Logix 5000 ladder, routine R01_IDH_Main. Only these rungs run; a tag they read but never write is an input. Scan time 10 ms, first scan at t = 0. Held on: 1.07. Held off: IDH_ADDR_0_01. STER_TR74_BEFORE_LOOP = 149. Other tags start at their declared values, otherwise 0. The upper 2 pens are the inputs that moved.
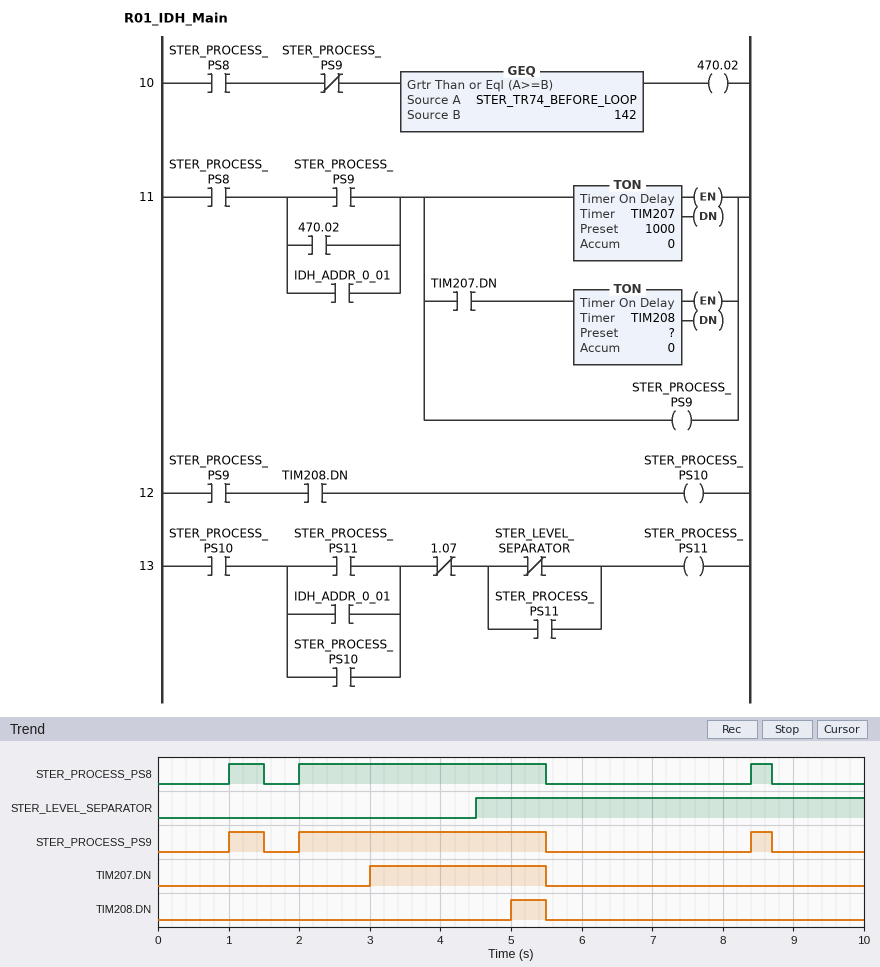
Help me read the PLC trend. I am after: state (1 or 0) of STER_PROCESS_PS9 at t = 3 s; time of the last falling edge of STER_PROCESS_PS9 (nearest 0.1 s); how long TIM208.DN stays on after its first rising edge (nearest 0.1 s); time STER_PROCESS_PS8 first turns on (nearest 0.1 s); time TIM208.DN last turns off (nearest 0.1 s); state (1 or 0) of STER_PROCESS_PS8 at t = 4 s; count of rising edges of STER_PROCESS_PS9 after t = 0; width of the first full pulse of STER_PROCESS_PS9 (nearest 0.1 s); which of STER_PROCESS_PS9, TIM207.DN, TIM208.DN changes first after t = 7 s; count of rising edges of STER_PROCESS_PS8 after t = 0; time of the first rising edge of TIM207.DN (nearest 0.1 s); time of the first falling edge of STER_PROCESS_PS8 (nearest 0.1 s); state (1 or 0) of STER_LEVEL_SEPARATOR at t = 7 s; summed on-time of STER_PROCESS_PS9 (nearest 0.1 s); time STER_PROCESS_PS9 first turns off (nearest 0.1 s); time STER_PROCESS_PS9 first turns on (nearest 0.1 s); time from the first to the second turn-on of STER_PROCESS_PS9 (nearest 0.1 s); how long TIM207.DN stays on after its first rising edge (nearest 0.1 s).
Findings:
1
8.7 s
0.5 s
1.0 s
5.5 s
1
3
0.5 s
STER_PROCESS_PS9
3
3.0 s
1.5 s
1
4.3 s
1.5 s
1.0 s
1.0 s
2.5 s
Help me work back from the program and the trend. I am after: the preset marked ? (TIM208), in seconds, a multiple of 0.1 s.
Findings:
2.0 s
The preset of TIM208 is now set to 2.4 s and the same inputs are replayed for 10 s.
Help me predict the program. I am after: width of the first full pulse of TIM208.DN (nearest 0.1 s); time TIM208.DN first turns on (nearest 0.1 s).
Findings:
0.1 s
5.4 s
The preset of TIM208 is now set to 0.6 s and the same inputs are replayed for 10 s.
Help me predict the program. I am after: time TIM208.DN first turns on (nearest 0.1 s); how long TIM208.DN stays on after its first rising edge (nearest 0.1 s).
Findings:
3.6 s
1.9 s
